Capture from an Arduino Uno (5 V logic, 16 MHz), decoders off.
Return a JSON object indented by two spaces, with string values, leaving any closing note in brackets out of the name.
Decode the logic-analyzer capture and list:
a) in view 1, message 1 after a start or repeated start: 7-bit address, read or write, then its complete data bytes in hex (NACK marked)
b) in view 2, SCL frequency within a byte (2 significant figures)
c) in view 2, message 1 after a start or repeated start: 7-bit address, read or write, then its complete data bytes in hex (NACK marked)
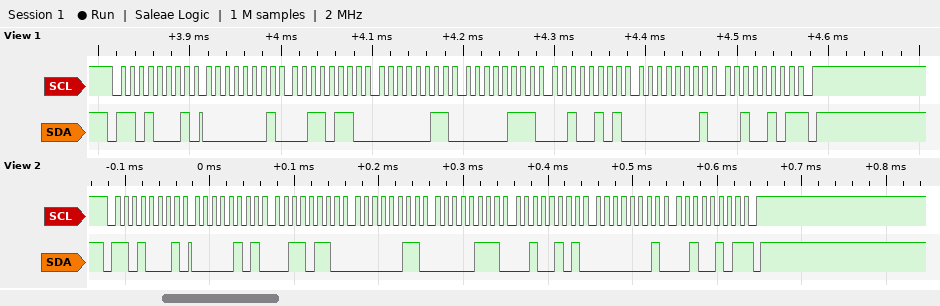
{
  "in view 1, message 1 after a start or repeated start: 7-bit address, read or write, then its complete data bytes in hex": "0x68 read: 01 36 03 07 25 01 25 NACK",
  "in view 2, SCL frequency within a byte": "100 kHz",
  "in view 2, message 1 after a start or repeated start: 7-bit address, read or write, then its complete data bytes in hex": "0x68 read: 05 36 03 07 25 01 25 NACK"
}
